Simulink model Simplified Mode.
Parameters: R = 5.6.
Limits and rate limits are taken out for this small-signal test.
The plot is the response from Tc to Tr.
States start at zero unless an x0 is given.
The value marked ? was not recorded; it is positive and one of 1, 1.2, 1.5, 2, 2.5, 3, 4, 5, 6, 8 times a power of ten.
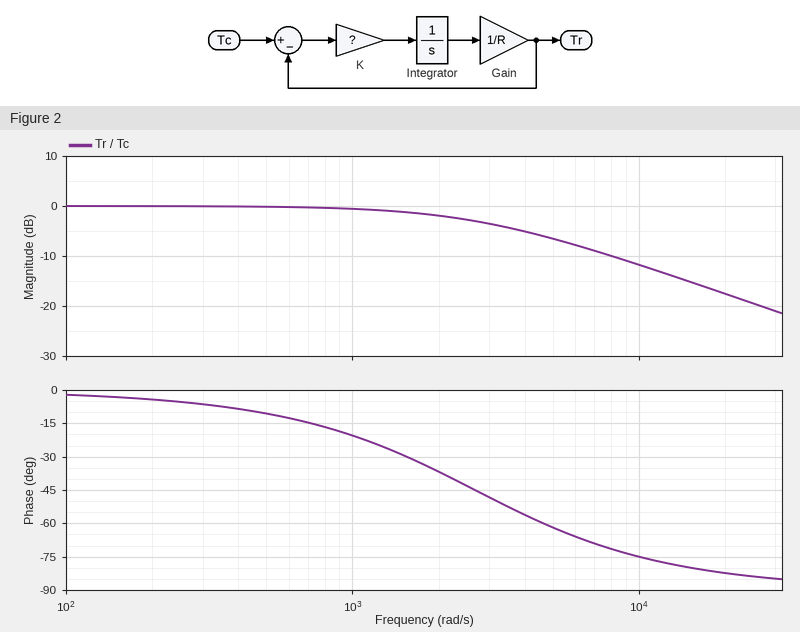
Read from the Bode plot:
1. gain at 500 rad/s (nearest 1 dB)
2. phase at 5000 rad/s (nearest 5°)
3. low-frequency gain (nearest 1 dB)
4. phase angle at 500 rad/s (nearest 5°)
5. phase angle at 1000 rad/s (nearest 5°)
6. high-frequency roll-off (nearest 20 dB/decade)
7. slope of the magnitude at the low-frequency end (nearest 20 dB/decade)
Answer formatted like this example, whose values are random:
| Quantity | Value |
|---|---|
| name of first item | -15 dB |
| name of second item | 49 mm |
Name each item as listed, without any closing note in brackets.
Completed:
| Quantity | Value |
|---|---|
| gain at 500 rad/s | 0 dB |
| phase at 5000 rad/s | -60° |
| low-frequency gain | 0 dB |
| phase angle at 500 rad/s | -10° |
| phase angle at 1000 rad/s | -20° |
| high-frequency roll-off | -20 dB/decade |
| slope of the magnitude at the low-frequency end | 0 dB/decade |
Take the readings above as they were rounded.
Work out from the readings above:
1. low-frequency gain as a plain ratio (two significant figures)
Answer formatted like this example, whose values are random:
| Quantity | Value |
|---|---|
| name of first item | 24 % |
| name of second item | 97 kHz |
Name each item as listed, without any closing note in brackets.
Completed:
| Quantity | Value |
|---|---|
| low-frequency gain as a plain ratio | 1.0 |
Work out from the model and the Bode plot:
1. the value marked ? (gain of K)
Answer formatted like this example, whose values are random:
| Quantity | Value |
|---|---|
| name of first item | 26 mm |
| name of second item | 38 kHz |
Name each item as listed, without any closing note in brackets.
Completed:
| Quantity | Value |
|---|---|
| the value marked ? | 15000 |
